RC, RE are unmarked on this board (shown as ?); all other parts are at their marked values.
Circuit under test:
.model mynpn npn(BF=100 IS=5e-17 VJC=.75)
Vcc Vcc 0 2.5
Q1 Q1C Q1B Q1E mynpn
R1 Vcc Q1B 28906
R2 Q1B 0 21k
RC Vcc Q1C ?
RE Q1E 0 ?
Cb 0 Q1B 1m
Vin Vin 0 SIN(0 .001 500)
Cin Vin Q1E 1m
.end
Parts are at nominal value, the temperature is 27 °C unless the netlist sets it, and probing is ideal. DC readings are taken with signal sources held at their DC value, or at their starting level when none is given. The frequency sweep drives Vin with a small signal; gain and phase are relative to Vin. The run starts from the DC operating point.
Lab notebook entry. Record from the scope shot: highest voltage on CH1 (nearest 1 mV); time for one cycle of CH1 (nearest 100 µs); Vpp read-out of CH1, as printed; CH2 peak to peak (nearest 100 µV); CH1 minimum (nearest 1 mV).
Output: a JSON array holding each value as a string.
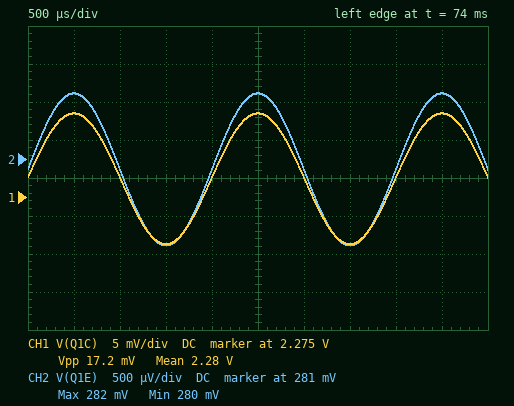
["2.286 V", "2.0 ms", "17.2 mV", "2.0 mV", "2.269 V"]
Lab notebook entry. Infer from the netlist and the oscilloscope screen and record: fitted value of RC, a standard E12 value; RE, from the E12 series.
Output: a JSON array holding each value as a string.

["1.2 kΩ", "1.5 kΩ"]
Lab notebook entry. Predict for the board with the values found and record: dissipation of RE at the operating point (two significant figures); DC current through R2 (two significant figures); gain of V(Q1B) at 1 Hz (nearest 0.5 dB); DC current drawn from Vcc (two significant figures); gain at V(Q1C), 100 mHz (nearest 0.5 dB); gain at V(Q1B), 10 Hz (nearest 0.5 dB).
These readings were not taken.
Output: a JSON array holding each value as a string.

["53 µW", "49 µA", "-43.0 dB", "240 µA", "-3.5 dB", "-59.0 dB"]
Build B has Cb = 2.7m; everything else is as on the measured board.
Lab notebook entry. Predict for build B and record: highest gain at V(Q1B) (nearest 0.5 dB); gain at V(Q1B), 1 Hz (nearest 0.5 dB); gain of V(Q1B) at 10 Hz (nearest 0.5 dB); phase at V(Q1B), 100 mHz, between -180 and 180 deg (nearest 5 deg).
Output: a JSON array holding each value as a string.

["-49.5 dB", "-51.5 dB", "-67.5 dB", "0 deg"]
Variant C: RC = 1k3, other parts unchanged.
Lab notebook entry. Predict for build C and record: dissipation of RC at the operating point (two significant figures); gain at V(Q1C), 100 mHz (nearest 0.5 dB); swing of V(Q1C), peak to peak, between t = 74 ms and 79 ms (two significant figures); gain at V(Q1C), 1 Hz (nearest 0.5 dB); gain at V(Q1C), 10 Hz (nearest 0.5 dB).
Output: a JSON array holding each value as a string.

["45 µW", "-2.5 dB", "19 mV", "15.0 dB", "19.5 dB"]
